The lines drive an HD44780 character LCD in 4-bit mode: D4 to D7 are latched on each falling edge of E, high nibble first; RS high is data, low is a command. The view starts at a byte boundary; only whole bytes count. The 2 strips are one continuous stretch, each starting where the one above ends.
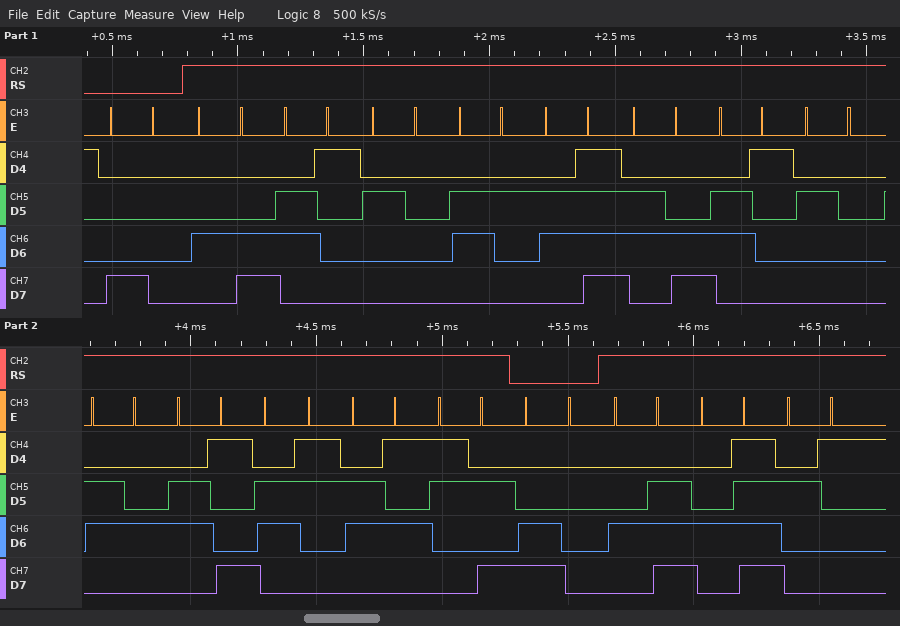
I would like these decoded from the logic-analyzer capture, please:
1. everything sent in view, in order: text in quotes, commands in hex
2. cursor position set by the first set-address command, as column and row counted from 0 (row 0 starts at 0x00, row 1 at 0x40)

0x80 "La bola dice:" 0xC0 "NO!"
column 0, row 0
